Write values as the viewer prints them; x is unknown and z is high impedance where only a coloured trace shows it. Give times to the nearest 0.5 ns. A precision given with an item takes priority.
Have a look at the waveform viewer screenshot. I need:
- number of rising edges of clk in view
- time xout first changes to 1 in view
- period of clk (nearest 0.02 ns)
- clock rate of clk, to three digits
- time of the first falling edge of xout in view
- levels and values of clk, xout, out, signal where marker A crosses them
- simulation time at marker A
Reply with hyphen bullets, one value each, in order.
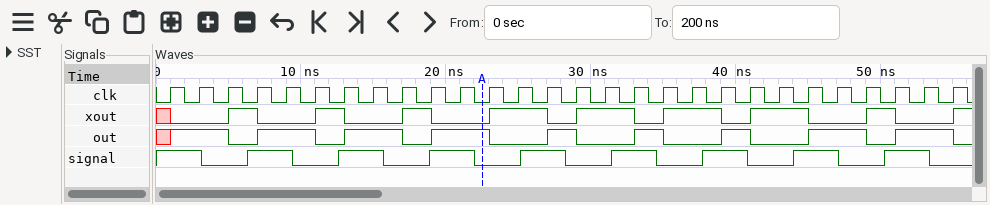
- 28
- 5 ns
- 2 ns
- 500 MHz
- 7 ns
- clk=0, xout=0, out=1, signal=0
- 22.5 ns
